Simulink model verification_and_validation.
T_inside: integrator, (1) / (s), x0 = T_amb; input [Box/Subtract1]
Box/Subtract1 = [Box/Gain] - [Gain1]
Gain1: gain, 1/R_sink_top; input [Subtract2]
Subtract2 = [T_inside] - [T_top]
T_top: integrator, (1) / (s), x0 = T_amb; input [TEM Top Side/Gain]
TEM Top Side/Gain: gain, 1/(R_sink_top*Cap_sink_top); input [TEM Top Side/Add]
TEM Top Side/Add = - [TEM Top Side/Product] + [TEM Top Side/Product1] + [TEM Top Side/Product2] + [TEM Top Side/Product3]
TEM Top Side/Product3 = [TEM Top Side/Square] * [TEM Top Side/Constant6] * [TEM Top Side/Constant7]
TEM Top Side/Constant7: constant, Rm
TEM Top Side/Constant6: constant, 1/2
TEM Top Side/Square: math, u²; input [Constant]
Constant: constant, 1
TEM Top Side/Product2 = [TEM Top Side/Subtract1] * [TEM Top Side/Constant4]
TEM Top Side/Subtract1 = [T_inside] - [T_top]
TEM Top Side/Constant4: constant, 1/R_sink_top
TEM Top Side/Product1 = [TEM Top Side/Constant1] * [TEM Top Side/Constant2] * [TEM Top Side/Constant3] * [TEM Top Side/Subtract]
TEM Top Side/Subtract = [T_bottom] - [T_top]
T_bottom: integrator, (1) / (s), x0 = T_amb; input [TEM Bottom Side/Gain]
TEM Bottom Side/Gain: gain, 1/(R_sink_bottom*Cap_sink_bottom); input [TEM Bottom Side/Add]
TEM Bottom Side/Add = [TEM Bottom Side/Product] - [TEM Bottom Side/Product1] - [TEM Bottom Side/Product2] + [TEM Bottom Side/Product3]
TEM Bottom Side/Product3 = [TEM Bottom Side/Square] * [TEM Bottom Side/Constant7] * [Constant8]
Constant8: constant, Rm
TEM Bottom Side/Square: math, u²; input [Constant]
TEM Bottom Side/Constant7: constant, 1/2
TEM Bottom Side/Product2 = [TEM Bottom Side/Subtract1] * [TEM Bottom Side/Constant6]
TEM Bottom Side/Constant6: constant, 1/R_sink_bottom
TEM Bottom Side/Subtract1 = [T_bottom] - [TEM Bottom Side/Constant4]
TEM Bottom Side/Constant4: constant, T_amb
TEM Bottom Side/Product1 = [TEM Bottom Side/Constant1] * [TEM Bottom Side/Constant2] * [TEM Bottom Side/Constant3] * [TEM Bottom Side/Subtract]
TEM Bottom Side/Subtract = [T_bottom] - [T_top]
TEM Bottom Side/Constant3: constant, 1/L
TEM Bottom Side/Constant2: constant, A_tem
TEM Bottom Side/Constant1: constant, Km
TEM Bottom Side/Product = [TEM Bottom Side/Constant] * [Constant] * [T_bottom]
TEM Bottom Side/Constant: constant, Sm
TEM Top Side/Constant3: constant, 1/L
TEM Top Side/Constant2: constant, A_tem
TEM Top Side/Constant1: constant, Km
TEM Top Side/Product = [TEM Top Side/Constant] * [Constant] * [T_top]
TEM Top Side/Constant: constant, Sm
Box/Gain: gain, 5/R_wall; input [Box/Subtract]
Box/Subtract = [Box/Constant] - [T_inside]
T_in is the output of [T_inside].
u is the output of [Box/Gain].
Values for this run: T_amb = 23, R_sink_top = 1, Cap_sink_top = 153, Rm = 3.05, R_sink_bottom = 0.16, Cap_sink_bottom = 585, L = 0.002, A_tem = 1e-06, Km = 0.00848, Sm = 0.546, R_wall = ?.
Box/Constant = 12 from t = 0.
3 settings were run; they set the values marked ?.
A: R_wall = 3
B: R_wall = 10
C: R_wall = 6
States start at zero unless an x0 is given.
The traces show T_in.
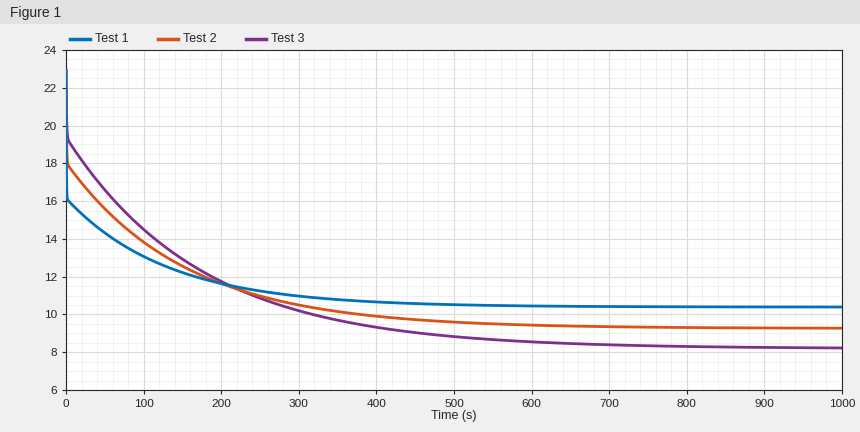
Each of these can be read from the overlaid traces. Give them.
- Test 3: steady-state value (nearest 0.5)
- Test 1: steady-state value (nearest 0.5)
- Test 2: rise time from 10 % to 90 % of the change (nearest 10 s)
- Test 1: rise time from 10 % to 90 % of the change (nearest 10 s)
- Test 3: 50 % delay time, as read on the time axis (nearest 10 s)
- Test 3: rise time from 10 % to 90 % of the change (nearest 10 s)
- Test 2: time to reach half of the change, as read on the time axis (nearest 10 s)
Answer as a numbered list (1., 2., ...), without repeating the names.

1. 8.0
2. 10.5
3. 280 s
4. 200 s
5. 70 s
6. 350 s
7. 40 s
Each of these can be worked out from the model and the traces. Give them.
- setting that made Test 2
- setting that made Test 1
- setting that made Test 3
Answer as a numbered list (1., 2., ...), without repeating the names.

1. C
2. A
3. B
